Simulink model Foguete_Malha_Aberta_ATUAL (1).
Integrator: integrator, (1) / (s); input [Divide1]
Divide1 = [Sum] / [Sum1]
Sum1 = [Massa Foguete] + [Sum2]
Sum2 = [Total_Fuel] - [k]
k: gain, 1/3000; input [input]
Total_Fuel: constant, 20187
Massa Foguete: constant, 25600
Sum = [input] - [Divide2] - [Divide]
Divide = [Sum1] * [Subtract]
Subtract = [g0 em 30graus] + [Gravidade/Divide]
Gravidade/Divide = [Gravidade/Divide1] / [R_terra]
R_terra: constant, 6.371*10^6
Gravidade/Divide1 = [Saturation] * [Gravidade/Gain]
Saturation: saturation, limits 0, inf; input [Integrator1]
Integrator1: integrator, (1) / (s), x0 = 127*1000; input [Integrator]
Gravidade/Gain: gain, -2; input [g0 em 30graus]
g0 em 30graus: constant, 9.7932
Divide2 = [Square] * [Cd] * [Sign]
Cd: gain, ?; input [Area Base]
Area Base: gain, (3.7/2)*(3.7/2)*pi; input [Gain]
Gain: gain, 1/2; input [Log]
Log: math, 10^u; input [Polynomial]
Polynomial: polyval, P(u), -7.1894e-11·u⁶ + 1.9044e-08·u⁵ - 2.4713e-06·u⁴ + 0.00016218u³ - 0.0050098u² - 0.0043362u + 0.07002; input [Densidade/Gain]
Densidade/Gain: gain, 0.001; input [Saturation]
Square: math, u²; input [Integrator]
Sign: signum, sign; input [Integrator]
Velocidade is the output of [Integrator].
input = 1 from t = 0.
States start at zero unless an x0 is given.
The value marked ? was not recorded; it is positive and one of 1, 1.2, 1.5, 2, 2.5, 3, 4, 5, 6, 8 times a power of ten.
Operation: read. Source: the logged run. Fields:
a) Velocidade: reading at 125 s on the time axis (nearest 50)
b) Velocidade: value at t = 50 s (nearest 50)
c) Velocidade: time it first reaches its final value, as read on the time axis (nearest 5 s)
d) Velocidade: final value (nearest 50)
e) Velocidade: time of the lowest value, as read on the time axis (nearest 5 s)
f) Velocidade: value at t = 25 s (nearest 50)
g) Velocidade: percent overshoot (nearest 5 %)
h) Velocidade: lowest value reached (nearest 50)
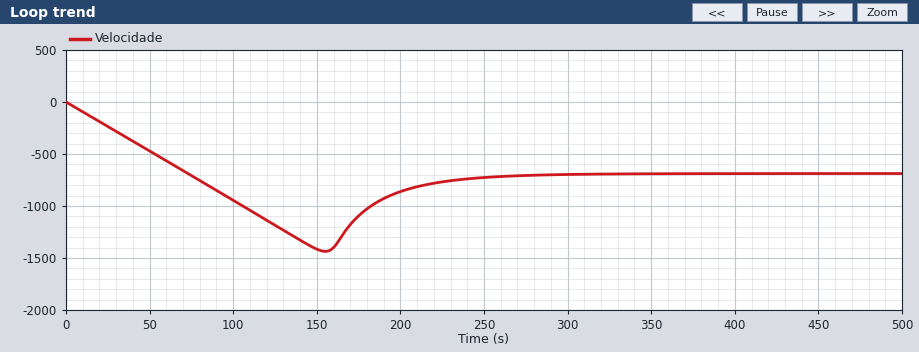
-1200
-450
75 s
-700
155 s
-250
110 %
-1450
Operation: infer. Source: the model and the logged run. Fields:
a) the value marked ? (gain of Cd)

0.15
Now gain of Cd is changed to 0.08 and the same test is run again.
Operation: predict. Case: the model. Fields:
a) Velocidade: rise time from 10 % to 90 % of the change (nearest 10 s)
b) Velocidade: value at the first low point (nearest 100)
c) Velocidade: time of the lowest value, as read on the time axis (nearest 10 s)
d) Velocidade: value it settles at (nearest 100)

80 s
-1500
160 s
-900
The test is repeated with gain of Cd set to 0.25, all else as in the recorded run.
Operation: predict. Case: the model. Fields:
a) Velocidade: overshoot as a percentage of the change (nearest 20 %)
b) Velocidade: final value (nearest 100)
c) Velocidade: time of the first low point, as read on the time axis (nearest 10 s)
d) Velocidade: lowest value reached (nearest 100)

160 %
-500
150 s
-1400
